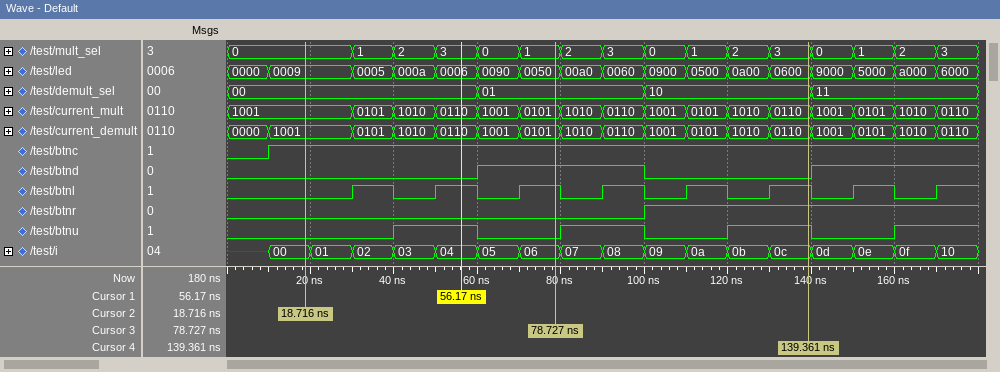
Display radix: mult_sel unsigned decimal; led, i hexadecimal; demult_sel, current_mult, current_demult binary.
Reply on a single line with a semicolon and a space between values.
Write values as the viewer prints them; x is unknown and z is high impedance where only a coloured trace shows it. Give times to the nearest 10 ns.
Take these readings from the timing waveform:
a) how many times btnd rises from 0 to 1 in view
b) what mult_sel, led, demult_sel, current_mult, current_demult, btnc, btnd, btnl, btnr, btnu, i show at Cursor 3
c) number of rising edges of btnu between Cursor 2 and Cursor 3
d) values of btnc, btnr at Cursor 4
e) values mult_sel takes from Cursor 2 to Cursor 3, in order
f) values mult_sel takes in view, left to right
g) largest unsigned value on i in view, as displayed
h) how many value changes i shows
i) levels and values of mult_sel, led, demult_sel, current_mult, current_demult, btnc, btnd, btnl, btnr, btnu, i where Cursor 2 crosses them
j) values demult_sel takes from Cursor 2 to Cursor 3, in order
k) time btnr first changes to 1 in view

2; mult_sel=1, led=0050, demult_sel=01, current_mult=0101, current_demult=0101, btnc=1, btnd=1, btnl=1, btnr=0, btnu=0, i=06; 1; btnc=1, btnr=1; 0, 1, 2, 3, 0, 1; 0, 1, 2, 3, 0, 1, 2, 3, 0, 1, 2, 3, 0, 1, 2, 3; 10; 17; mult_sel=0, led=0009, demult_sel=00, current_mult=1001, current_demult=1001, btnc=1, btnd=0, btnl=0, btnr=0, btnu=0, i=00; 00, 01; 100 ns
